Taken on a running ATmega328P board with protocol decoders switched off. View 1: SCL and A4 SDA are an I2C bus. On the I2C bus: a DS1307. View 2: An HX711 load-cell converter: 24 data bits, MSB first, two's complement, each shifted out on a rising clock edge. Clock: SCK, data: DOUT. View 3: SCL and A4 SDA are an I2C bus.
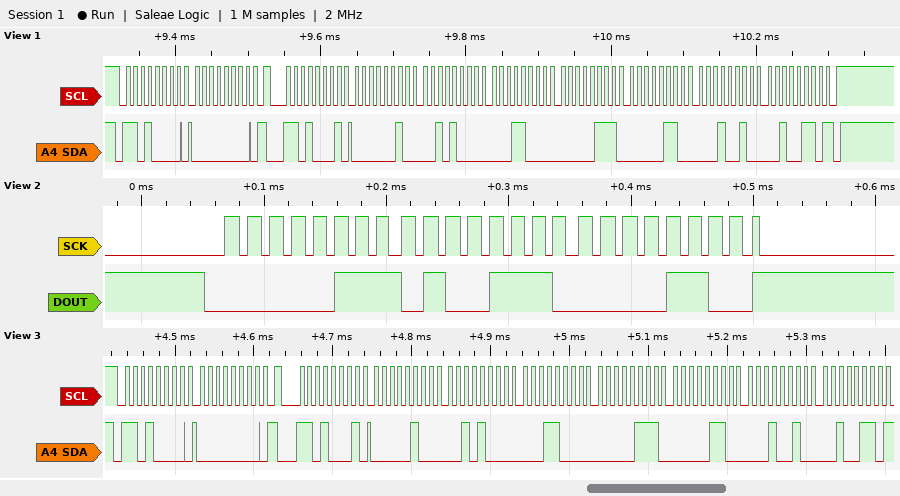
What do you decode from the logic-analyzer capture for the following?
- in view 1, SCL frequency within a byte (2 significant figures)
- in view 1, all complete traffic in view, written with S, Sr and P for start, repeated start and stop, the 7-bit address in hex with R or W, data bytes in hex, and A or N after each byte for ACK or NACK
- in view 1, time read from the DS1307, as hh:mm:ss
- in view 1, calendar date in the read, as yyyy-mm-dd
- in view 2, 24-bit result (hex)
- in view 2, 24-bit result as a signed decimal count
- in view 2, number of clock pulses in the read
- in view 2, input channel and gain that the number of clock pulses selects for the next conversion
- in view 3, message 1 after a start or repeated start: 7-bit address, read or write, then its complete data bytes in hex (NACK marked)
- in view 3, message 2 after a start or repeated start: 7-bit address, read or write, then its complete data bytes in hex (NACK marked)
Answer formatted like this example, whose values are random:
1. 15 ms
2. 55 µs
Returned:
1. 100 kHz
2. S 68W A 00 A Sr 68R A 02 A 28 A 18 A 07 A 06 A 12 A 26 N P
3. 18:28:02
4. 2026-12-06
5. 0x074E0C
6. 478732
7. 25
8. channel A, gain 128
9. 0x68 write: 00
10. 0x68 read: 04 28 18 07 06 12 26 NACK
